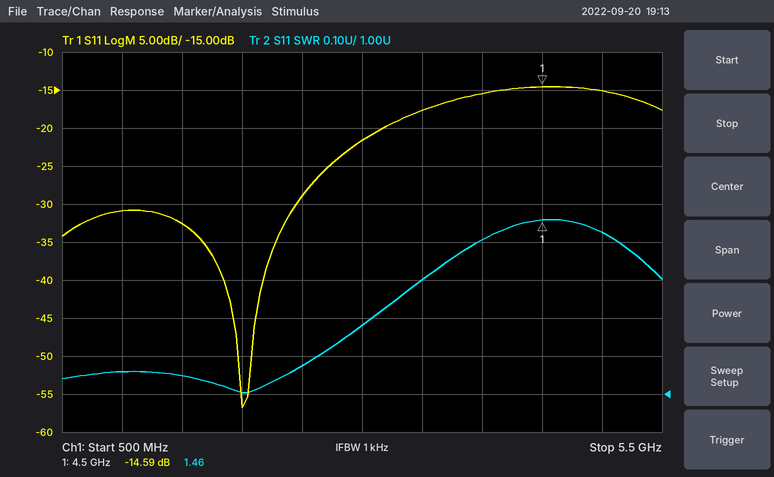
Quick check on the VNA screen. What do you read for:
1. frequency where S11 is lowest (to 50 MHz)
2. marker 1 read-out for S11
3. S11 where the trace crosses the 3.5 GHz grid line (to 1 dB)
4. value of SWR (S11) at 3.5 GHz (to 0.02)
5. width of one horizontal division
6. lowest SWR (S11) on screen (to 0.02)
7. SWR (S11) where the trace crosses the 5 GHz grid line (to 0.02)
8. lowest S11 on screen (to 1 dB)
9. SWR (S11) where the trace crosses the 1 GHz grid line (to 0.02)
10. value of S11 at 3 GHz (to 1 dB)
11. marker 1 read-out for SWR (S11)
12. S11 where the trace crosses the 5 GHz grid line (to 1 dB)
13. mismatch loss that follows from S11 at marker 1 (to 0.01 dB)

2.00 GHz
-14.59 dB
-18 dB
1.30
500 MHz
1.00
1.42
-57 dB
1.06
-22 dB
1.46
-15 dB
0.15 dB
